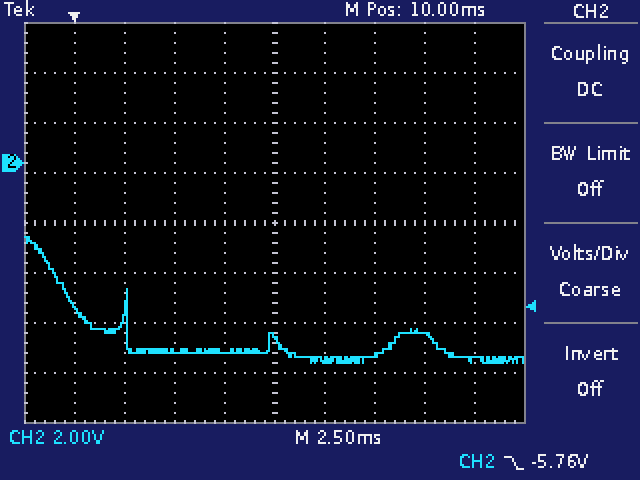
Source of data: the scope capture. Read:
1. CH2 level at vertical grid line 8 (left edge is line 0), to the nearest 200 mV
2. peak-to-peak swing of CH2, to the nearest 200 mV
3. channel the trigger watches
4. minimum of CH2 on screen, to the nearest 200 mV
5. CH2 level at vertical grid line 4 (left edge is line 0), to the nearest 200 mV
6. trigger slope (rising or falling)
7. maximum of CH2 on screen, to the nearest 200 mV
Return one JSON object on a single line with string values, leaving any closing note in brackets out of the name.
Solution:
{"CH2 level at vertical grid line 8 (left edge is line 0), to the nearest 200 mV": "-6.8 V", "peak-to-peak swing of CH2, to the nearest 200 mV": "5.0 V", "channel the trigger watches": "CH2", "minimum of CH2 on screen, to the nearest 200 mV": "-8.0 V", "CH2 level at vertical grid line 4 (left edge is line 0), to the nearest 200 mV": "-7.6 V", "trigger slope": "falling", "maximum of CH2 on screen, to the nearest 200 mV": "-3.0 V"}
